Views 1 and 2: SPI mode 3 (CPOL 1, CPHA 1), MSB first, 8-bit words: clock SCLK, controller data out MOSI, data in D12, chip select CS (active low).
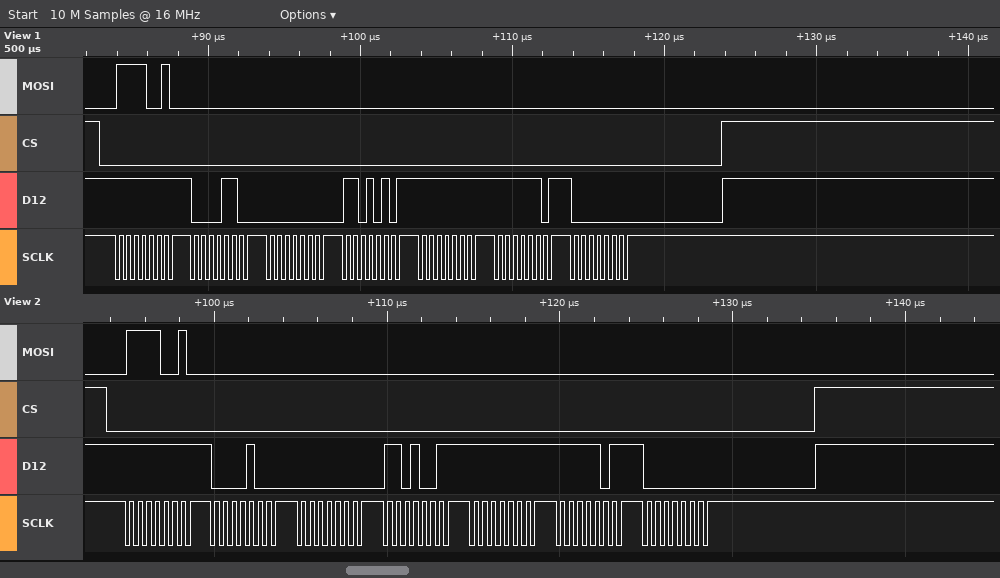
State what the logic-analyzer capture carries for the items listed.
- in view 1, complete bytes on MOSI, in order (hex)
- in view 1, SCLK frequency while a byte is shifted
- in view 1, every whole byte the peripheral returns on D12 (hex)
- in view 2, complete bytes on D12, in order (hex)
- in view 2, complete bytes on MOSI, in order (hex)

0xF2 0x00 0x00 0x00 0x00 0x00 0x00
2 MHz
0xFF 0x0C 0x00 0xD5 0xFF 0xFD 0x00
FF 08 00 D3 FF FB 00
F2 00 00 00 00 00 00
